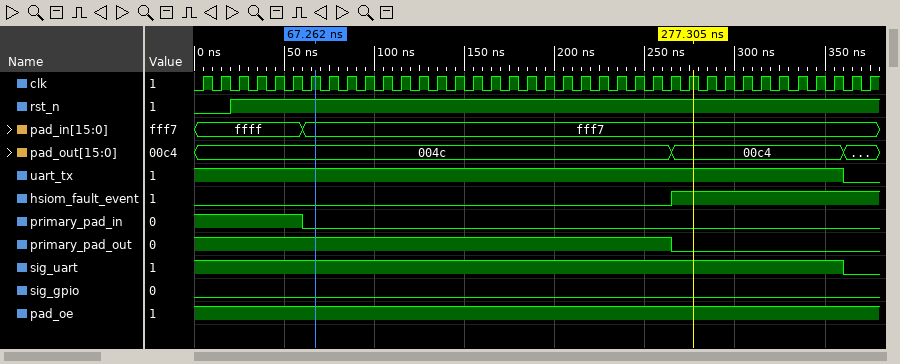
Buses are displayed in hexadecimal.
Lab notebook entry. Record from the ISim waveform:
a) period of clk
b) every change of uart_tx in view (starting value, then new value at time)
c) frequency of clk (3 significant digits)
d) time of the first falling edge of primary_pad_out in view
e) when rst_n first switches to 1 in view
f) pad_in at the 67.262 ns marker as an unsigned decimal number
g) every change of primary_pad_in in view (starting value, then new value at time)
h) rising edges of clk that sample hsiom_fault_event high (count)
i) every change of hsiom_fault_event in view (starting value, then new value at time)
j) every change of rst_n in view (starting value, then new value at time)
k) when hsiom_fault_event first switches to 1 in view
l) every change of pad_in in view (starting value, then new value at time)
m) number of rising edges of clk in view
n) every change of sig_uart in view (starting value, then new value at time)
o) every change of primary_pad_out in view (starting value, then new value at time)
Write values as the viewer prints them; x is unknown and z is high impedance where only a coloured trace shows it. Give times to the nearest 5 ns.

10 ns
1, 0 at 360 ns
100 MHz
265 ns
20 ns
65527
1, 0 at 60 ns
11
0, 1 at 265 ns
0, 1 at 20 ns
265 ns
ffff, fff7 at 60 ns
38
1, 0 at 360 ns
1, 0 at 265 ns
